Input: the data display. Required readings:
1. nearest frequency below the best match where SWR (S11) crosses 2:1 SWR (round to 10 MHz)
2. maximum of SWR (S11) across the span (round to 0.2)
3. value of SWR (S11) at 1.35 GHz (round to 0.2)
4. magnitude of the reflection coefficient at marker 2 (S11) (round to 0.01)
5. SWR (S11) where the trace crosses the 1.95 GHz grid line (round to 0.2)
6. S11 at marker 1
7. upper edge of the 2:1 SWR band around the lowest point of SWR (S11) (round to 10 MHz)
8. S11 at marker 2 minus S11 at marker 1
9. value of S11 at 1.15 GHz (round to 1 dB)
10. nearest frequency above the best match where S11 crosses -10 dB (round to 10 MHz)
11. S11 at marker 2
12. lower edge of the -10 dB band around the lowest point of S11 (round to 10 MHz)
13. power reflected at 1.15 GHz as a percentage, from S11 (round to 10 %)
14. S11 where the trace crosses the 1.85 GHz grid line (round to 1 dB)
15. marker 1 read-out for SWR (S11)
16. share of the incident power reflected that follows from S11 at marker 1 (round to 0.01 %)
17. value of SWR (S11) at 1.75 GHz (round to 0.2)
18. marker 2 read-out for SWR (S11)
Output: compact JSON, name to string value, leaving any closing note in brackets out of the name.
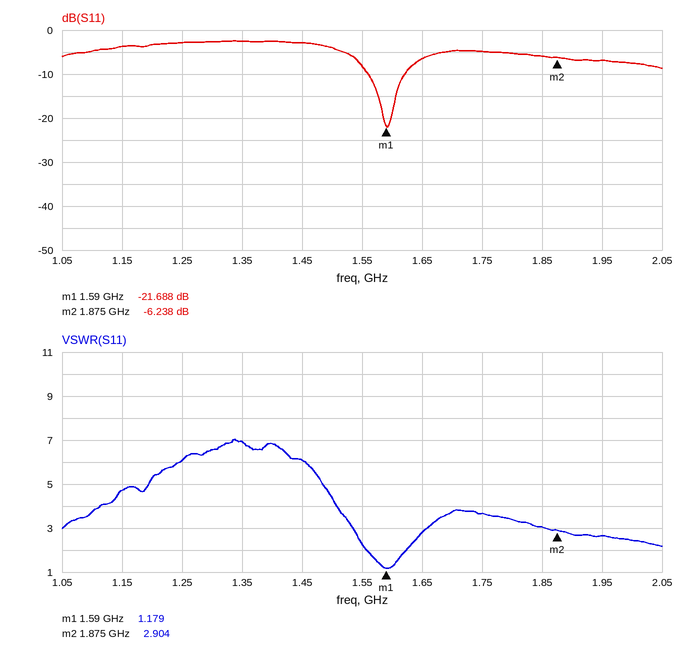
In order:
{"nearest frequency below the best match where SWR (S11) crosses 2:1 SWR": "1.56 GHz", "maximum of SWR (S11) across the span": "7.0", "value of SWR (S11) at 1.35 GHz": "7.0", "magnitude of the reflection coefficient at marker 2 (S11)": "0.49", "SWR (S11) where the trace crosses the 1.95 GHz grid line": "2.6", "S11 at marker 1": "-21.688 dB", "upper edge of the 2:1 SWR band around the lowest point of SWR (S11)": "1.62 GHz", "S11 at marker 2 minus S11 at marker 1": "15.450 dB", "value of S11 at 1.15 GHz": "-4 dB", "nearest frequency above the best match where S11 crosses -10 dB": "1.62 GHz", "S11 at marker 2": "-6.238 dB", "lower edge of the -10 dB band around the lowest point of S11": "1.56 GHz", "power reflected at 1.15 GHz as a percentage, from S11": "40 %", "S11 where the trace crosses the 1.85 GHz grid line": "-6 dB", "marker 1 read-out for SWR": "1.179", "share of the incident power reflected that follows from S11 at marker 1": "0.68 %", "value of SWR (S11) at 1.75 GHz": "3.6", "marker 2 read-out for SWR": "2.904"}
